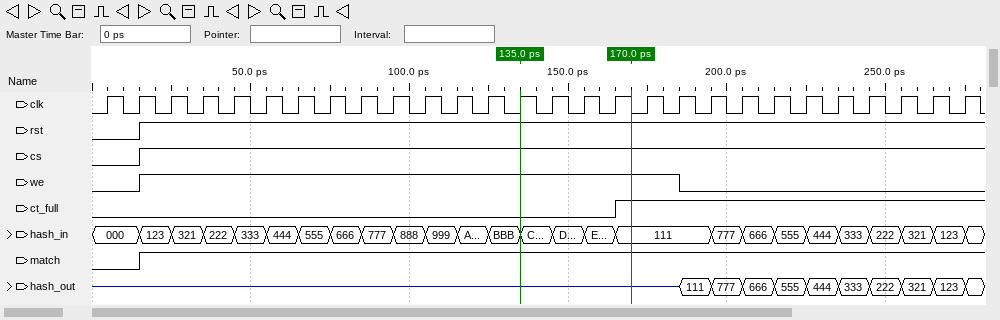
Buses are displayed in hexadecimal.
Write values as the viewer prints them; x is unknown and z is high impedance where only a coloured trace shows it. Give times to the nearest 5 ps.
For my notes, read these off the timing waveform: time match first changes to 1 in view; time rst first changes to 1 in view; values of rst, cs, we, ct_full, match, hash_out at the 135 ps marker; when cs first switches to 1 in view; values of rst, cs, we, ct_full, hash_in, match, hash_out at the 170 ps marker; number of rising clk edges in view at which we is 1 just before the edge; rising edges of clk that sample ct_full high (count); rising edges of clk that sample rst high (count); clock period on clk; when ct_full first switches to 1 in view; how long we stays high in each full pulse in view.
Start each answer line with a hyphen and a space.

- 15 ps
- 15 ps
- rst=1, cs=1, we=1, ct_full=0, match=1, hash_out=z
- 15 ps
- rst=1, cs=1, we=1, ct_full=1, hash_in=111, match=1, hash_out=z
- 17
- 11
- 26
- 10 ps
- 165 ps
- 170 ps
